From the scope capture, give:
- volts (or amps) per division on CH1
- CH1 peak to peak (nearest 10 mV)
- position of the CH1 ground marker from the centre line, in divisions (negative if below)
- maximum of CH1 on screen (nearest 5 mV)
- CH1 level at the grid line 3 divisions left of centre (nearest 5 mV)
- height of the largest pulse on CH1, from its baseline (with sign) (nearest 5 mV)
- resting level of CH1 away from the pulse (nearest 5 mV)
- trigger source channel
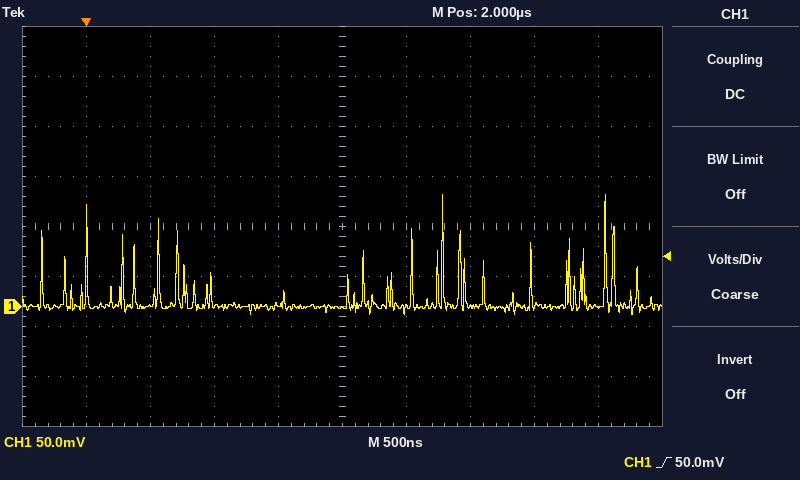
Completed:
50 mV
120 mV
-1.6 div
110 mV
0 mV
+110 mV
0 mV
CH1
